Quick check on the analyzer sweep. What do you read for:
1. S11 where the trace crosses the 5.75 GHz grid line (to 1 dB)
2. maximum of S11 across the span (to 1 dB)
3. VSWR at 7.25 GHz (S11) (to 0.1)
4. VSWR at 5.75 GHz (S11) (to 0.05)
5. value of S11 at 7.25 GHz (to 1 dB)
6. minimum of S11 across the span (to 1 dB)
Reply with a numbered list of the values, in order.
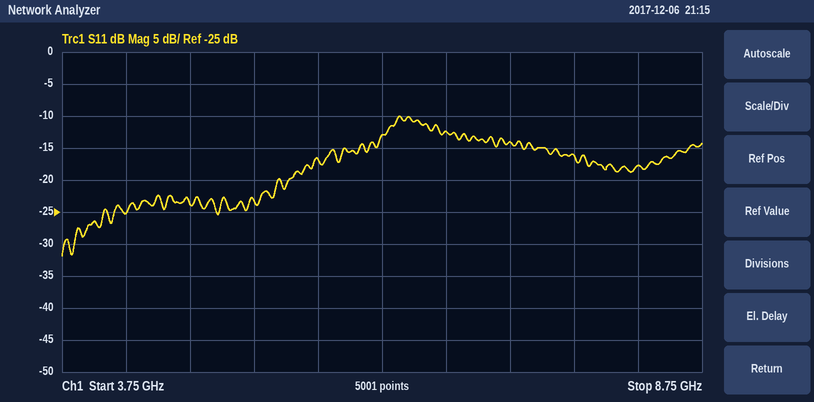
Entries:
1. -17 dB
2. -10 dB
3. 1.5
4. 1.35
5. -14 dB
6. -32 dB
